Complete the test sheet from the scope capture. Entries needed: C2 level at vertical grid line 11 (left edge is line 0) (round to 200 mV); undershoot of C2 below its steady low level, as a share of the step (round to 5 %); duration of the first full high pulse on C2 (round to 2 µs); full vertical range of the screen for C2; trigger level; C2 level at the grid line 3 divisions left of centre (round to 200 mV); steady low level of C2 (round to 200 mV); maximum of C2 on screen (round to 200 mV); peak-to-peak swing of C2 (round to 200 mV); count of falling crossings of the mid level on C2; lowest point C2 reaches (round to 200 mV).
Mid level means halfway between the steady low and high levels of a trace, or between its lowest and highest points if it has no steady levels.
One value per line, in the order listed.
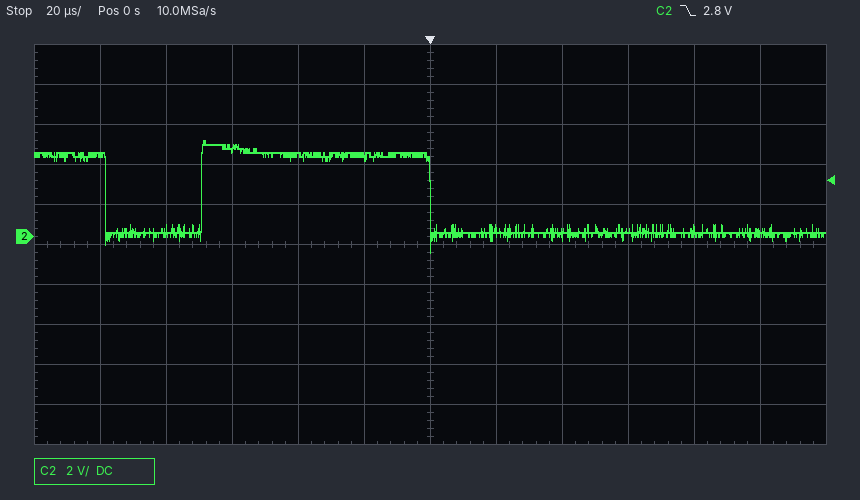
200 mV
25 %
70 µs
20 V
2.8 V
4.4 V
200 mV
4.8 V
5.6 V
2
-800 mV
